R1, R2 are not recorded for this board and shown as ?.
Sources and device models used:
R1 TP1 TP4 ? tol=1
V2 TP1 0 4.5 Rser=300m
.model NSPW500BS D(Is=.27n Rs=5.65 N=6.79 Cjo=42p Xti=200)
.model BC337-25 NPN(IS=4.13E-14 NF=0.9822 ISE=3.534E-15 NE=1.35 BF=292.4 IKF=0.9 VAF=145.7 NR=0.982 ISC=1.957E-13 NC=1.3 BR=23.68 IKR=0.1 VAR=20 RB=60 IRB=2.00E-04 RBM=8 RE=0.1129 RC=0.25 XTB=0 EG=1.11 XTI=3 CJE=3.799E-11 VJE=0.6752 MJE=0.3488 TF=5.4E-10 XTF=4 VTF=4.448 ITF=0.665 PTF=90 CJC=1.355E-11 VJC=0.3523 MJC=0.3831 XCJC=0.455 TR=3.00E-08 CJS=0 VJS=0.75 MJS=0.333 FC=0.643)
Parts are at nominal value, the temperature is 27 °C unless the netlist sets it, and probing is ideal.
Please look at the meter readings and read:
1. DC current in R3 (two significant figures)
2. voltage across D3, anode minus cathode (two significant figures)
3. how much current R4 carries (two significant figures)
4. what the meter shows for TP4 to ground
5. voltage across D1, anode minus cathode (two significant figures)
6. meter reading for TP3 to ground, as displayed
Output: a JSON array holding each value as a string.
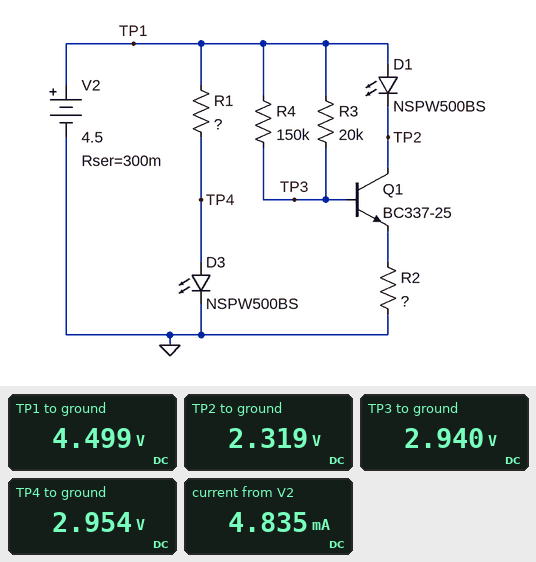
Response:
["78 µA", "3.0 V", "10 µA", "2.954 V", "2.2 V", "2.940 V"]
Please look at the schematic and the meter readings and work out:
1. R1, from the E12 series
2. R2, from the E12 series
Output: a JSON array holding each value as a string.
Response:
["330 Ω", "15 kΩ"]
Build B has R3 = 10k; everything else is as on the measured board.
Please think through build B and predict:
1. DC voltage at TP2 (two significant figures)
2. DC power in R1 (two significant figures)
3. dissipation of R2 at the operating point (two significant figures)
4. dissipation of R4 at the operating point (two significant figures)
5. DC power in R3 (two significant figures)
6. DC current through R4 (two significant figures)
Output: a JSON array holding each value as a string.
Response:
["2.5 V", "7.2 mW", "420 µW", "12 µW", "180 µW", "9.0 µA"]
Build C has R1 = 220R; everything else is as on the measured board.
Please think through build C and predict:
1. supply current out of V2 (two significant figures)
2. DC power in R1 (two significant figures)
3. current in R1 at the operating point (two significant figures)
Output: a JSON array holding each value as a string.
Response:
["6.8 mA", "9.8 mW", "6.7 mA"]
